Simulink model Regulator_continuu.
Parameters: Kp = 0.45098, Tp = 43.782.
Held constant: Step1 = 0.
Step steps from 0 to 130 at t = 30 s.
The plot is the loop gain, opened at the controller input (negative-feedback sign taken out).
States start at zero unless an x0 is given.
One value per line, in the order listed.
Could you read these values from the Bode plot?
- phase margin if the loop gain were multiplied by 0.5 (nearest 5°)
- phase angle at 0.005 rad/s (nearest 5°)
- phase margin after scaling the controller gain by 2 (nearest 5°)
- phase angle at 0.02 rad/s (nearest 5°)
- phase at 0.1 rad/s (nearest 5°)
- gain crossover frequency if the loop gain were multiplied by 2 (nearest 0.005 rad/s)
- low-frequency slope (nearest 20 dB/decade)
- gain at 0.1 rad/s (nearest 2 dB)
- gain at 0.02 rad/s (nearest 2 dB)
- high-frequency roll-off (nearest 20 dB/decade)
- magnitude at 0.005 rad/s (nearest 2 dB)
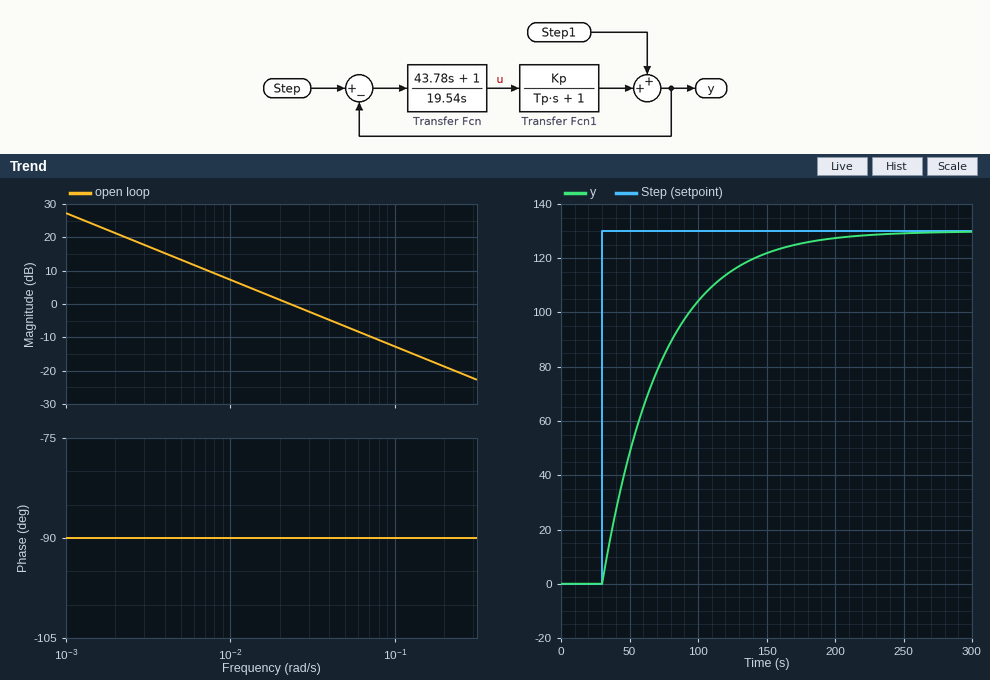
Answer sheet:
90°
-90°
90°
-90°
-90°
0.045 rad/s
-20 dB/decade
-12 dB
2 dB
-20 dB/decade
14 dB
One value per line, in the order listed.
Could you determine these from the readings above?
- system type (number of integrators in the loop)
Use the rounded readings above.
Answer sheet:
1
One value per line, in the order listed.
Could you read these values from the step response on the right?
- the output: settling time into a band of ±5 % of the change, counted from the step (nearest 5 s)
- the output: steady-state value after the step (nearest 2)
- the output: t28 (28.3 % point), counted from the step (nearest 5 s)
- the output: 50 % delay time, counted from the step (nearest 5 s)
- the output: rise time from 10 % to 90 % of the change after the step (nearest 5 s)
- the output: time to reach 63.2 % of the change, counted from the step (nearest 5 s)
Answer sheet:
130 s
130
15 s
30 s
95 s
45 s
